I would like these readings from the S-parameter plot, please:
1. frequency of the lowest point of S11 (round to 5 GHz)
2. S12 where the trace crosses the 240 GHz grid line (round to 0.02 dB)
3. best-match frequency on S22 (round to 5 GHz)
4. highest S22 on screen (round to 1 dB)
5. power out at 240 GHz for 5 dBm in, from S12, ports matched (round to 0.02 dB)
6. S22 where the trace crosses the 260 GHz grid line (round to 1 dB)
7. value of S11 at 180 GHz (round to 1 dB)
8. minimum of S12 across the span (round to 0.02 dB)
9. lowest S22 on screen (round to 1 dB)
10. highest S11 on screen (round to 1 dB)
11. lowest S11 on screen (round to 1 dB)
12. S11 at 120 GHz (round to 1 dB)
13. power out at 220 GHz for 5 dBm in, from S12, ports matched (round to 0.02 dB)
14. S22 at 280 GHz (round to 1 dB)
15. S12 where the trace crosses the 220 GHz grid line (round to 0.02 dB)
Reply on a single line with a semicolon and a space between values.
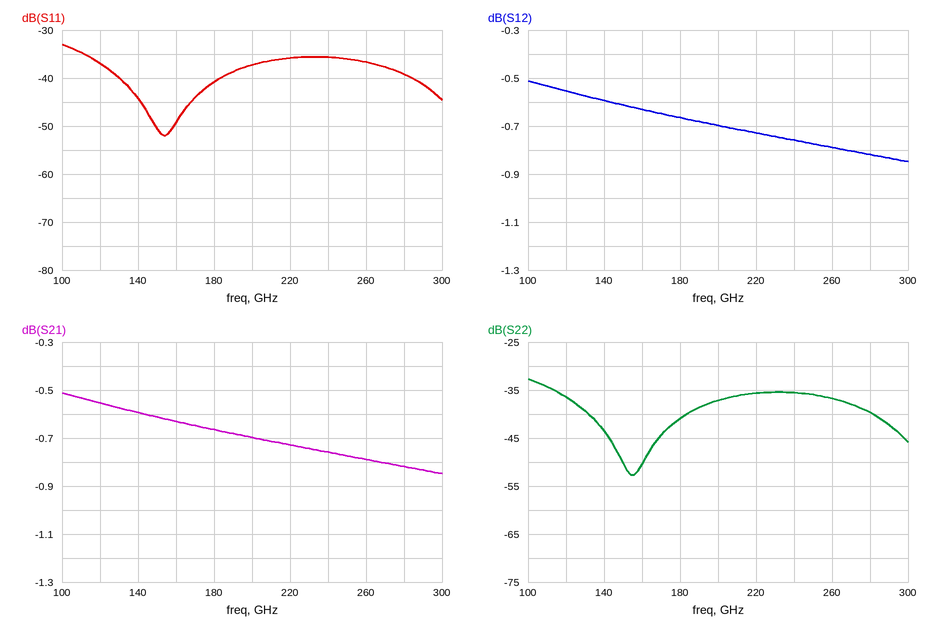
155 GHz; -0.76 dB; 155 GHz; -33 dB; 4.24 dBm; -37 dB; -41 dB; -0.84 dB; -53 dB; -33 dB; -52 dB; -37 dB; 4.28 dBm; -40 dB; -0.72 dB
